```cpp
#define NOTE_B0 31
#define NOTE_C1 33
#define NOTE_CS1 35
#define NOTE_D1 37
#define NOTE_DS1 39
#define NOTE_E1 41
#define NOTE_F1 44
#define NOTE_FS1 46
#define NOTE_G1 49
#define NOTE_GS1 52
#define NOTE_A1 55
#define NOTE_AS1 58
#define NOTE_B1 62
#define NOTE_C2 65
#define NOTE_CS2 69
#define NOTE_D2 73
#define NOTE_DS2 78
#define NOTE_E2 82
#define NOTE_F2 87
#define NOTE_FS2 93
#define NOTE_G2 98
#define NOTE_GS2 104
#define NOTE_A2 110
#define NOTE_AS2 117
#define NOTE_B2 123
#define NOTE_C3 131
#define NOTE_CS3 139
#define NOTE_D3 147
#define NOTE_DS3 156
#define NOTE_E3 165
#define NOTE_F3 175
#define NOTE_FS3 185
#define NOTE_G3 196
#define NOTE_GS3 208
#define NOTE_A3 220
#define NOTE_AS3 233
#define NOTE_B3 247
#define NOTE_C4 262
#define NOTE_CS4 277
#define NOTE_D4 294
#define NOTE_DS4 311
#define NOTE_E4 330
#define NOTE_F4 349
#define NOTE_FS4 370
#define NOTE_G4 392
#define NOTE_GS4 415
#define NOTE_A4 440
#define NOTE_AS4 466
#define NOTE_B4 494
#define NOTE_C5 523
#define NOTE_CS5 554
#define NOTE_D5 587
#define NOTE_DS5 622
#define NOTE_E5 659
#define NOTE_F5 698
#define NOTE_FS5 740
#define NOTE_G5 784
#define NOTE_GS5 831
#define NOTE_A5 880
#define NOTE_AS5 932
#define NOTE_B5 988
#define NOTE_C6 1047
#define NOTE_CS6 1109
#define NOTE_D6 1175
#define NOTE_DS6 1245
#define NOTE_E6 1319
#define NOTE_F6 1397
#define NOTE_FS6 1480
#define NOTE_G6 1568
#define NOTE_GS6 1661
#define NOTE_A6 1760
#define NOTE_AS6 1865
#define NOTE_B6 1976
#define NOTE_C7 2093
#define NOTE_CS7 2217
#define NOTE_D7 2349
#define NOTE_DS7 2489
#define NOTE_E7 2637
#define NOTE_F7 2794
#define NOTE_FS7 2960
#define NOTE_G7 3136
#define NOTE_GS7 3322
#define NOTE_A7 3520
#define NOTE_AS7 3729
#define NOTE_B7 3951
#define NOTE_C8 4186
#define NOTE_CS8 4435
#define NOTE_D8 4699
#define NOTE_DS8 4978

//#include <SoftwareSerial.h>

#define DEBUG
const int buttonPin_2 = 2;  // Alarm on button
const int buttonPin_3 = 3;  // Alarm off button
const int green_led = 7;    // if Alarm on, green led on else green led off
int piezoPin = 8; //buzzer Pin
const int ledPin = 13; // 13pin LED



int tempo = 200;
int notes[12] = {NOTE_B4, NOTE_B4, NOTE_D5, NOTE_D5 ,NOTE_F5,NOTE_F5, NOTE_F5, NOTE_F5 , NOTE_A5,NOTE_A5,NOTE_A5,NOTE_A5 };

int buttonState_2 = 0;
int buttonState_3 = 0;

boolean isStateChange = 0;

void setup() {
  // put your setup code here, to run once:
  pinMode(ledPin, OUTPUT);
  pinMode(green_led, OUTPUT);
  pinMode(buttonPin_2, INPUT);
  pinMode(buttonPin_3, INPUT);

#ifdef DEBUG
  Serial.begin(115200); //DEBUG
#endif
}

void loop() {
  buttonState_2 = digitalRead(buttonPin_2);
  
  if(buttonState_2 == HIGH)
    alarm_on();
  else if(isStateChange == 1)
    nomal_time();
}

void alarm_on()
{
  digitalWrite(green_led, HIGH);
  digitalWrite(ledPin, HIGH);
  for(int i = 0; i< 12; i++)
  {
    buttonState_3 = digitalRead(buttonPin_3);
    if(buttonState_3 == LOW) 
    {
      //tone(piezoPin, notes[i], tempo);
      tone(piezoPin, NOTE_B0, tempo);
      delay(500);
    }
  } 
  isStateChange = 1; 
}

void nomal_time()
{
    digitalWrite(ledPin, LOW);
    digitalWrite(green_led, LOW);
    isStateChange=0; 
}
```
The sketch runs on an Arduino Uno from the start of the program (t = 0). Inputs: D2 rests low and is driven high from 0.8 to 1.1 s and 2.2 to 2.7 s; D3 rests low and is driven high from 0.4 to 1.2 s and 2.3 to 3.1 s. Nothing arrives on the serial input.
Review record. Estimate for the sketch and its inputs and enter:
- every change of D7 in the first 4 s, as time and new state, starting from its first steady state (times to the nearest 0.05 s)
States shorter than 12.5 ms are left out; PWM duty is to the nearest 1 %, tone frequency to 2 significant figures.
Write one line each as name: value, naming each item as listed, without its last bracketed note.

every change of D7 in the first 4 s, as time and new state, starting from its first steady state: 0 s low; 0.8 s high; 1.1 s low; 2.2 s high; 2.7 s low
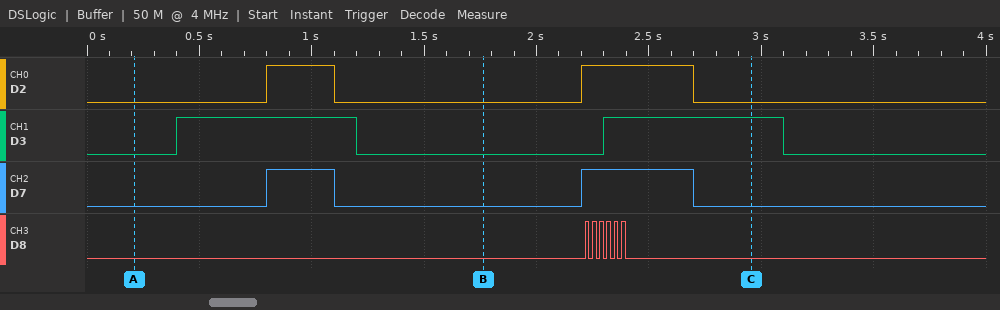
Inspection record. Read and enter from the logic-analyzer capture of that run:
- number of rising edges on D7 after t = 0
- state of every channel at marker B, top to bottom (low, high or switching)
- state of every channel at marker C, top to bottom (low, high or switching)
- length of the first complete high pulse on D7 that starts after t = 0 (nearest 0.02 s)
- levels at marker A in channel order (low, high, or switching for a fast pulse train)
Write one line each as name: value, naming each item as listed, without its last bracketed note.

number of rising edges on D7 after t = 0: 2
state of every channel at marker B, top to bottom: D2 low, D3 low, D7 low, D8 low
state of every channel at marker C, top to bottom: D2 low, D3 high, D7 low, D8 low
length of the first complete high pulse on D7 that starts after t = 0: 0.30 s
levels at marker A in channel order: D2 low, D3 low, D7 low, D8 low
